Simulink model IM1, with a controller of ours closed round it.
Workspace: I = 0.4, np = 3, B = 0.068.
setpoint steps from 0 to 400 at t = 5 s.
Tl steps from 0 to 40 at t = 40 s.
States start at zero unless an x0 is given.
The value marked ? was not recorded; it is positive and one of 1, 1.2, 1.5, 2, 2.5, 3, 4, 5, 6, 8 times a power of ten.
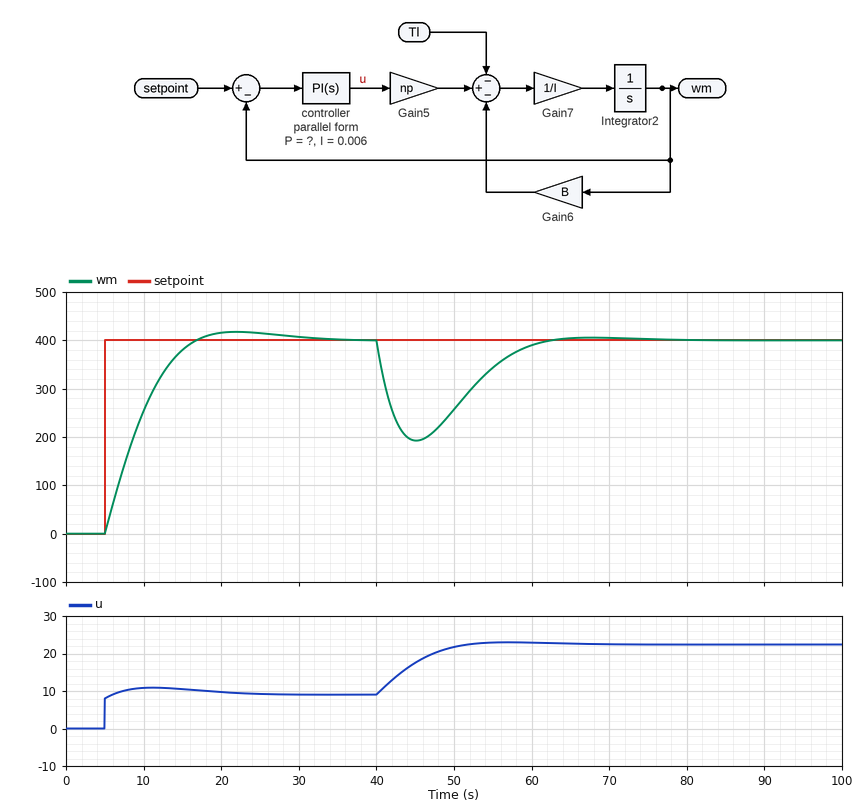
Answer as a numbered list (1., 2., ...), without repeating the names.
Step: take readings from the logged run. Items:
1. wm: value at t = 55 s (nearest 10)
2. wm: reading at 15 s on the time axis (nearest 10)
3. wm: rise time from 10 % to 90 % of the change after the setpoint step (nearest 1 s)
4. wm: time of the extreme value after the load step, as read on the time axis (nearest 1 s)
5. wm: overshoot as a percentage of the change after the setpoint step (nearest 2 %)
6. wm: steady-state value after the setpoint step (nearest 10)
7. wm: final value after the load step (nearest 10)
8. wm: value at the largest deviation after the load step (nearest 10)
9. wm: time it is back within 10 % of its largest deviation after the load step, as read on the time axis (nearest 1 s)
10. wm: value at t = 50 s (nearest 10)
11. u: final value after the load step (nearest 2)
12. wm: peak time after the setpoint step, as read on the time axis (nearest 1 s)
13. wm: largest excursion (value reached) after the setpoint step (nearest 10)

1. 340
2. 380
3. 8 s
4. 45 s
5. 4 %
6. 400
7. 400
8. 190
9. 58 s
10. 260
11. 22
12. 22 s
13. 420
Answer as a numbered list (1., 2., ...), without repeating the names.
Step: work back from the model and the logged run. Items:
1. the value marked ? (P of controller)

1. 0.02
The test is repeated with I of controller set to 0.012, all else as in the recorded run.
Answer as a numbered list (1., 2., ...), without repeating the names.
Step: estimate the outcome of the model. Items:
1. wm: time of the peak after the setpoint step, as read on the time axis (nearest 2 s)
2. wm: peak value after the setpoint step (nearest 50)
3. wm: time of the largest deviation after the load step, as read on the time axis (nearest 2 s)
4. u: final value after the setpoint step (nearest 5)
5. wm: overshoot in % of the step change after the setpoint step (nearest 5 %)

1. 16 s
2. 450
3. 44 s
4. 10
5. 15 %
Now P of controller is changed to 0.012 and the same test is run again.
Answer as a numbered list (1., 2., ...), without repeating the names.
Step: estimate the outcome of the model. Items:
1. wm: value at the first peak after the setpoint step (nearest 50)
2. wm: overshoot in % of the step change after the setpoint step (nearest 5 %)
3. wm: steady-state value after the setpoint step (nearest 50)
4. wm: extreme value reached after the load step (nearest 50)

1. 450
2. 10 %
3. 400
4. 150
